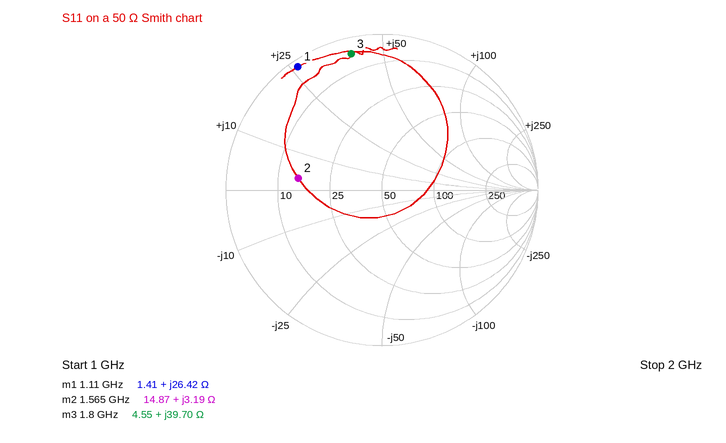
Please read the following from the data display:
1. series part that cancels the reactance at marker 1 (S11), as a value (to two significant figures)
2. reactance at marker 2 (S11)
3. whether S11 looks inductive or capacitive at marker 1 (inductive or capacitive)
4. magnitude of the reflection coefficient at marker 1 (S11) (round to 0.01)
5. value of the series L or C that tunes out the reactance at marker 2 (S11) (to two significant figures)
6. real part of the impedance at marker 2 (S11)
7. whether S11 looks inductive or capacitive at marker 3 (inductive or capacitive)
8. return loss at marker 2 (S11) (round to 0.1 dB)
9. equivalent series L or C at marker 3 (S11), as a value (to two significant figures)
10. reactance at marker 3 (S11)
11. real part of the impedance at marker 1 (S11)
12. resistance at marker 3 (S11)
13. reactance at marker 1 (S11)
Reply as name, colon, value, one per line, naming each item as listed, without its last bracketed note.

series part that cancels the reactance at marker 1 (S11), as a value: 5.4 pF
reactance at marker 2: +3.19 Ω
whether S11 looks inductive or capacitive at marker 1: inductive
magnitude of the reflection coefficient at marker 1 (S11): 0.96
value of the series L or C that tunes out the reactance at marker 2 (S11): 32 pF
real part of the impedance at marker 2: 14.87 Ω
whether S11 looks inductive or capacitive at marker 3: inductive
return loss at marker 2 (S11): 5.3 dB
equivalent series L or C at marker 3 (S11), as a value: 3.5 nH
reactance at marker 3: +39.70 Ω
real part of the impedance at marker 1: 1.41 Ω
resistance at marker 3: 4.55 Ω
reactance at marker 1: +26.42 Ω
